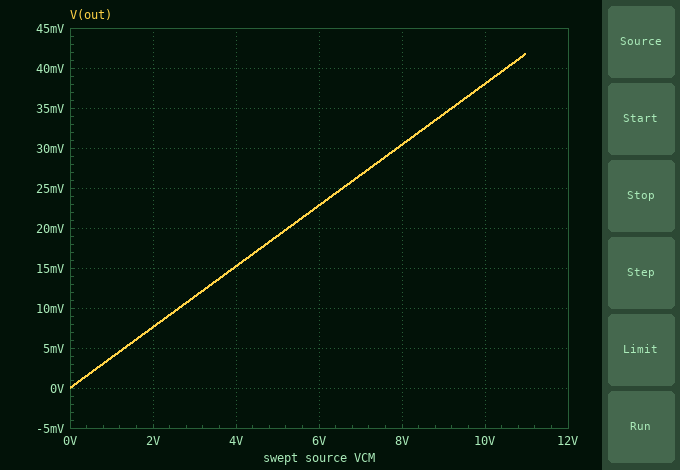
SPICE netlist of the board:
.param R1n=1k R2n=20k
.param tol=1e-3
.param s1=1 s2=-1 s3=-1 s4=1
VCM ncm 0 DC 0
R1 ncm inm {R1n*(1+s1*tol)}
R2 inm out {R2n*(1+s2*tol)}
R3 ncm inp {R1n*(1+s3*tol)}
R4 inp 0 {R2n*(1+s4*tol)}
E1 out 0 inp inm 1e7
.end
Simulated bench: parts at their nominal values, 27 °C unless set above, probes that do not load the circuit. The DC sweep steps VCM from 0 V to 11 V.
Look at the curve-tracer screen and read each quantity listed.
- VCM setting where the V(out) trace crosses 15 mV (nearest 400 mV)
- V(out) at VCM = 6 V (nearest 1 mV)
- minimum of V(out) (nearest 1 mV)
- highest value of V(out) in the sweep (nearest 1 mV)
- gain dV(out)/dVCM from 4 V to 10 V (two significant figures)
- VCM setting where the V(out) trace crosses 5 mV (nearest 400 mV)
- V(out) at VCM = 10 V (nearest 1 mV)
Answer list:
4.0 V
23 mV
0 V
42 mV
0.0038 V/V
1.2 V
38 mV
